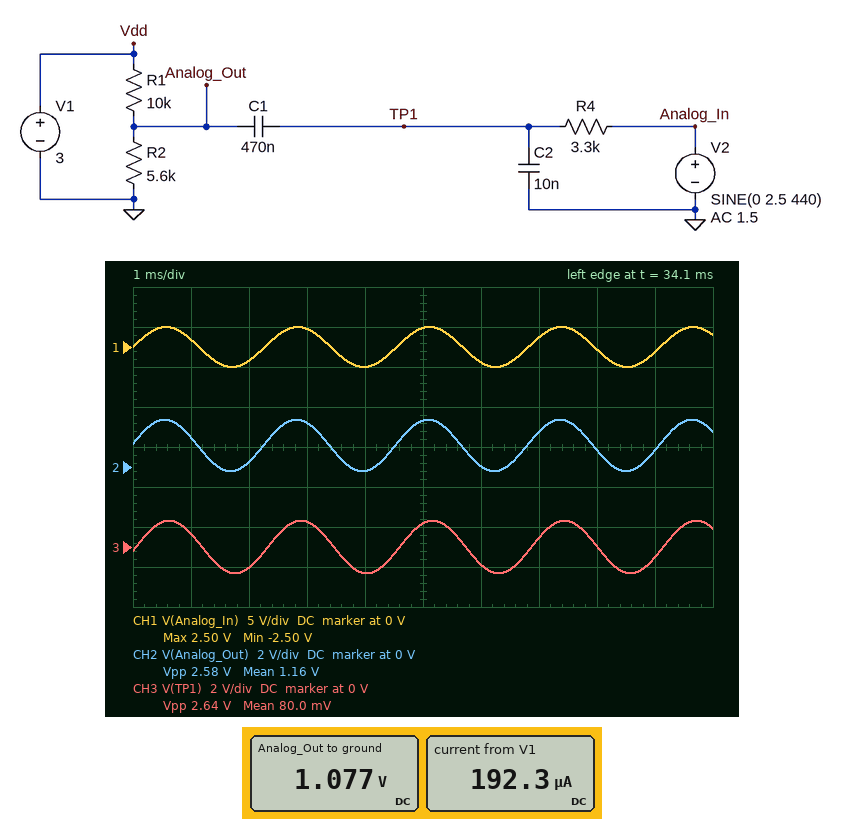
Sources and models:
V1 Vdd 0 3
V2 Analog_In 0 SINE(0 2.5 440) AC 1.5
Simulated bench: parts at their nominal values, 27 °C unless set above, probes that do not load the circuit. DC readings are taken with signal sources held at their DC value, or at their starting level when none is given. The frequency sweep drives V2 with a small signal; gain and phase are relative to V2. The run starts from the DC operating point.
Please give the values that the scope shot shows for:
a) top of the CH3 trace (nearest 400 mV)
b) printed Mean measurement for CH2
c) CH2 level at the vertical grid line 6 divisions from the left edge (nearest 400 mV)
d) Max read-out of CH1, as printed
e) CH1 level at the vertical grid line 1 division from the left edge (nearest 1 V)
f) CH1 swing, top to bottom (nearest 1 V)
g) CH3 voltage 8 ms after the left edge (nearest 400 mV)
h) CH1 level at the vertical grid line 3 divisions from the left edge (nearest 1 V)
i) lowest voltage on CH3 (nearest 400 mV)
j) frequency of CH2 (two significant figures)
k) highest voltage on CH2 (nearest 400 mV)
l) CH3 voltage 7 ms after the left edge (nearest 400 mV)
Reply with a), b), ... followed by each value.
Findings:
a) 1.2 V
b) 1.16 V
c) 0 V
d) 2.50 V
e) 1 V
f) 5 V
g) 0 V
h) 2 V
i) -1.2 V
j) 440 Hz
k) 2.4 V
l) 400 mV
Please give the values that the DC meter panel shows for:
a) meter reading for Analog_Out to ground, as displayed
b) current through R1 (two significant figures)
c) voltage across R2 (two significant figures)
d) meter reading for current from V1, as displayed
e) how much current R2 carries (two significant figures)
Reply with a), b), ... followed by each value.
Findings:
a) 1.077 V
b) 190 µA
c) 1.1 V
d) 192.3 µA
e) 190 µA
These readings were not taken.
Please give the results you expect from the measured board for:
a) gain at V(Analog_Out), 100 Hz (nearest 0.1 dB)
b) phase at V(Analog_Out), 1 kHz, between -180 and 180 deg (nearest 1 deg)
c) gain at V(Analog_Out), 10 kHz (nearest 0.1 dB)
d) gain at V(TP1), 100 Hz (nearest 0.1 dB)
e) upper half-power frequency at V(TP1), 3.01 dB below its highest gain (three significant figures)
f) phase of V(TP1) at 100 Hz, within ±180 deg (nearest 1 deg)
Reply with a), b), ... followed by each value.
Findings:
a) -6.6 dB
b) -3 deg
c) -9.0 dB
d) -3.9 dB
e) 71.9 Hz
f) -18 deg
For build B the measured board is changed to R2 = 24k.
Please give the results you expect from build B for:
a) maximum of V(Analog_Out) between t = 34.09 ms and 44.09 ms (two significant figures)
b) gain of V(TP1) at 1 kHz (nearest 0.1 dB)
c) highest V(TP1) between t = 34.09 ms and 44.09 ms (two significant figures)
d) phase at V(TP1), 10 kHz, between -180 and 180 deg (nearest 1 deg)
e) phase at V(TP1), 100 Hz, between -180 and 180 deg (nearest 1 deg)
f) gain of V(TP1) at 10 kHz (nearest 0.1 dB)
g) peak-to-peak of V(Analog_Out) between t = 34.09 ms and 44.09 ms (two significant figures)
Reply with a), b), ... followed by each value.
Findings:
a) 3.8 V
b) -3.4 dB
c) 1.7 V
d) -55 deg
e) -8 deg
f) -8.1 dB
g) 3.4 V
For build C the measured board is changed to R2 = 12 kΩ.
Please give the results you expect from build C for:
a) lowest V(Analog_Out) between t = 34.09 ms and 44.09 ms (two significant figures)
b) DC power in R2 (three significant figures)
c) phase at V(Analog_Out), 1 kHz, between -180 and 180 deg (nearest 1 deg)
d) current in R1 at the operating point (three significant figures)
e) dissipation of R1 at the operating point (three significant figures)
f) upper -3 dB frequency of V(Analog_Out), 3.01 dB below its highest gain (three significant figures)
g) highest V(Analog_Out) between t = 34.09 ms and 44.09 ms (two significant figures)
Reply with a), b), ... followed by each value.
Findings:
a) 92 mV
b) 223 µW
c) -5 deg
d) 136 µA
e) 186 µW
f) 7.84 kHz
g) 3.2 V
